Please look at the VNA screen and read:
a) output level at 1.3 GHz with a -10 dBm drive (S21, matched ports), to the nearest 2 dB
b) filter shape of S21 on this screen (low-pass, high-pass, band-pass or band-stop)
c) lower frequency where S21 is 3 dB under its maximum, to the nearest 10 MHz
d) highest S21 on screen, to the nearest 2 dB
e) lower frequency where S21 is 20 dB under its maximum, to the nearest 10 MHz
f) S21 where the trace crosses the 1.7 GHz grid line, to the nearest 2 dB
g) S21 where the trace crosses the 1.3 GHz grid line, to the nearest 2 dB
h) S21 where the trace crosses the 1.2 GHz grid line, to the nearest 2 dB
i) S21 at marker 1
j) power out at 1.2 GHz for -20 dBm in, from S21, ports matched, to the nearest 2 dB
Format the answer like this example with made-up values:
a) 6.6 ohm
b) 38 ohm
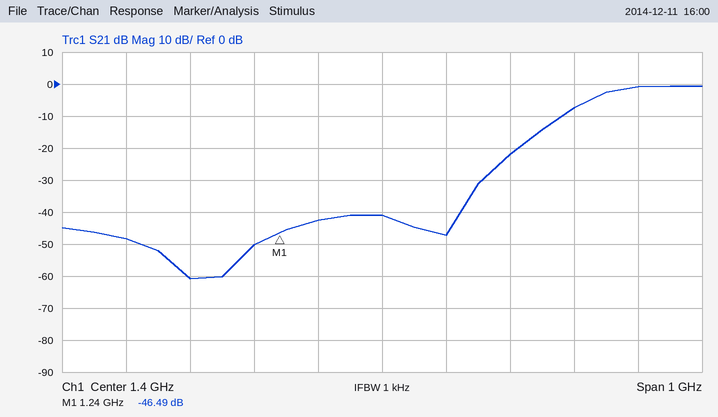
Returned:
a) -52 dBm
b) high-pass
c) 1.74 GHz
d) 0 dB
e) 1.61 GHz
f) -8 dB
g) -42 dB
h) -50 dB
i) -46.49 dB
j) -70 dBm
